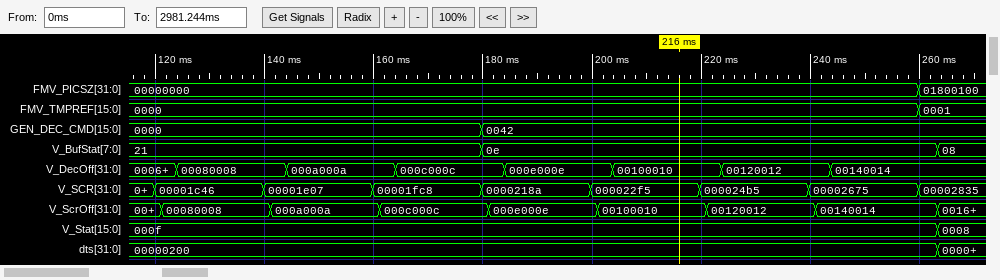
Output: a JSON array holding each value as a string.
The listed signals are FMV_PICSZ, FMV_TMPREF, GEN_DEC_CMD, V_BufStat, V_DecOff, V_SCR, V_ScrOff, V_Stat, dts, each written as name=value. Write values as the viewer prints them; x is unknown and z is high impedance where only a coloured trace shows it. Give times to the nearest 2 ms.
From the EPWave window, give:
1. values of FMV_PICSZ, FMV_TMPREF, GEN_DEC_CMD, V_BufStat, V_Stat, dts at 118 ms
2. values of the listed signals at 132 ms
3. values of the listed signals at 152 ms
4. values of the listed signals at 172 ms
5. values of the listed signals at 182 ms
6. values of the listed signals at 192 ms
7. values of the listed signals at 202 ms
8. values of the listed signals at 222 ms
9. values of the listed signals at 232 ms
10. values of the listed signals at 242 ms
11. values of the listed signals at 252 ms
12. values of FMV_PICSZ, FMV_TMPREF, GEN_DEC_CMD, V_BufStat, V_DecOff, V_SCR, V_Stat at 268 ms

["FMV_PICSZ=00000000, FMV_TMPREF=0000, GEN_DEC_CMD=0000, V_BufStat=21, V_Stat=000f, dts=00000200", "FMV_PICSZ=00000000, FMV_TMPREF=0000, GEN_DEC_CMD=0000, V_BufStat=21, V_DecOff=00080008, V_SCR=00001c46, V_ScrOff=00080008, V_Stat=000f, dts=00000200", "FMV_PICSZ=00000000, FMV_TMPREF=0000, GEN_DEC_CMD=0000, V_BufStat=21, V_DecOff=000a000a, V_SCR=00001e07, V_ScrOff=000a000a, V_Stat=000f, dts=00000200", "FMV_PICSZ=00000000, FMV_TMPREF=0000, GEN_DEC_CMD=0000, V_BufStat=21, V_DecOff=000c000c, V_SCR=00001fc8, V_ScrOff=000c000c, V_Stat=000f, dts=00000200", "FMV_PICSZ=00000000, FMV_TMPREF=0000, GEN_DEC_CMD=0042, V_BufStat=0e, V_DecOff=000c000c, V_SCR=0000218a, V_ScrOff=000e000e, V_Stat=000f, dts=00000200", "FMV_PICSZ=00000000, FMV_TMPREF=0000, GEN_DEC_CMD=0042, V_BufStat=0e, V_DecOff=000e000e, V_SCR=0000218a, V_ScrOff=000e000e, V_Stat=000f, dts=00000200", "FMV_PICSZ=00000000, FMV_TMPREF=0000, GEN_DEC_CMD=0042, V_BufStat=0e, V_DecOff=000e000e, V_SCR=000022f5, V_ScrOff=00100010, V_Stat=000f, dts=00000200", "FMV_PICSZ=00000000, FMV_TMPREF=0000, GEN_DEC_CMD=0042, V_BufStat=0e, V_DecOff=00100010, V_SCR=000024b5, V_ScrOff=00120012, V_Stat=000f, dts=00000200", "FMV_PICSZ=00000000, FMV_TMPREF=0000, GEN_DEC_CMD=0042, V_BufStat=0e, V_DecOff=00120012, V_SCR=000024b5, V_ScrOff=00120012, V_Stat=000f, dts=00000200", "FMV_PICSZ=00000000, FMV_TMPREF=0000, GEN_DEC_CMD=0042, V_BufStat=0e, V_DecOff=00120012, V_SCR=00002675, V_ScrOff=00140014, V_Stat=000f, dts=00000200", "FMV_PICSZ=00000000, FMV_TMPREF=0000, GEN_DEC_CMD=0042, V_BufStat=0e, V_DecOff=00140014, V_SCR=00002675, V_ScrOff=00140014, V_Stat=000f, dts=00000200", "FMV_PICSZ=01800100, FMV_TMPREF=0001, GEN_DEC_CMD=0042, V_BufStat=08, V_DecOff=00140014, V_SCR=00002835, V_Stat=0008"]
